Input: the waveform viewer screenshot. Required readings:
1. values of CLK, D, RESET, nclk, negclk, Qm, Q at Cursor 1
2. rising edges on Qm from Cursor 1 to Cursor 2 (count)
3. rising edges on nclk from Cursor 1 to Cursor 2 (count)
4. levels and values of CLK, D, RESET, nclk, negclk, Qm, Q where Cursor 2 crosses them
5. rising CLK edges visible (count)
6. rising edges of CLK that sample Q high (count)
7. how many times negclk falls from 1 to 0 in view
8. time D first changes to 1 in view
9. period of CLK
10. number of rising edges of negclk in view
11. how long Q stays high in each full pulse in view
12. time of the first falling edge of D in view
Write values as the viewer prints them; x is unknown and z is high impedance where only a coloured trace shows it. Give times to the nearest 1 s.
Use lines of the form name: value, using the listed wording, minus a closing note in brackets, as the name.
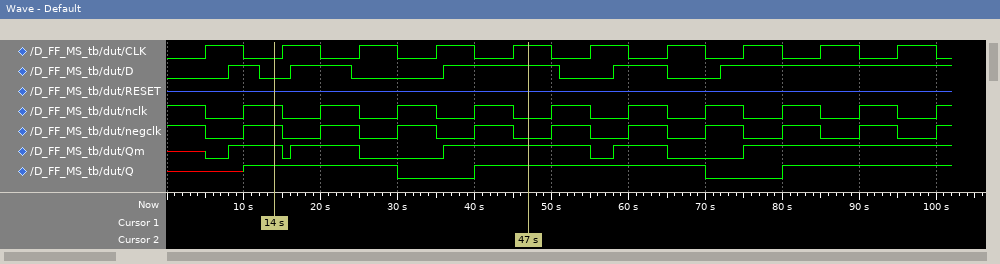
values of CLK, D, RESET, nclk, negclk, Qm, Q at Cursor 1: CLK=0, D=0, RESET=z, nclk=1, negclk=1, Qm=1, Q=1
rising edges on Qm from Cursor 1 to Cursor 2: 2
rising edges on nclk from Cursor 1 to Cursor 2: 3
levels and values of CLK, D, RESET, nclk, negclk, Qm, Q where Cursor 2 crosses them: CLK=1, D=1, RESET=z, nclk=0, negclk=0, Qm=1, Q=1
rising CLK edges visible: 10
rising edges of CLK that sample Q high: 7
how many times negclk falls from 1 to 0 in view: 10
time D first changes to 1 in view: 8 s
period of CLK: 10 s
number of rising edges of negclk in view: 10
how long Q stays high in each full pulse in view: 30 s
time of the first falling edge of D in view: 12 s
